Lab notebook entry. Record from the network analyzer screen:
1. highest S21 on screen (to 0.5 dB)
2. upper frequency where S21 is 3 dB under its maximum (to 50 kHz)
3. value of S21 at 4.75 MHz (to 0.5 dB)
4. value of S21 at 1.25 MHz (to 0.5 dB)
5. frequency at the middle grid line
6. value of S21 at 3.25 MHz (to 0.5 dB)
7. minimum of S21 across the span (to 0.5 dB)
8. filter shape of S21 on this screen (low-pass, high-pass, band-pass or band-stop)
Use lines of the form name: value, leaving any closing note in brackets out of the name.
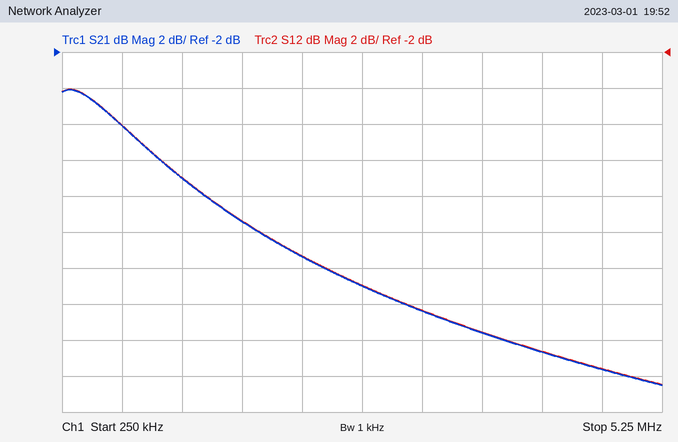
highest S21 on screen: -4.0 dB
upper frequency where S21 is 3 dB under its maximum: 900 kHz
value of S21 at 4.75 MHz: -19.5 dB
value of S21 at 1.25 MHz: -9.0 dB
frequency at the middle grid line: 2.75 MHz
value of S21 at 3.25 MHz: -16.5 dB
minimum of S21 across the span: -20.5 dB
filter shape of S21 on this screen: low-pass
